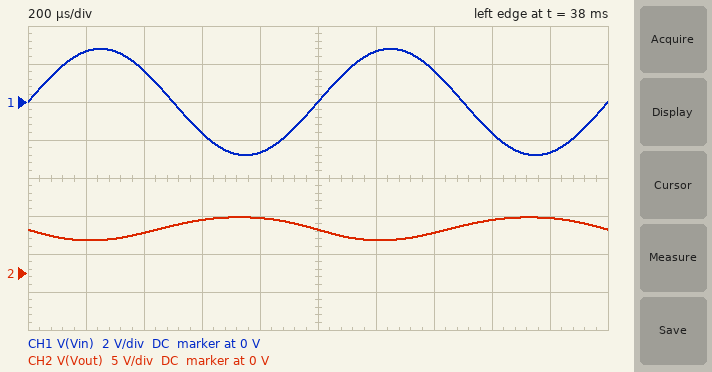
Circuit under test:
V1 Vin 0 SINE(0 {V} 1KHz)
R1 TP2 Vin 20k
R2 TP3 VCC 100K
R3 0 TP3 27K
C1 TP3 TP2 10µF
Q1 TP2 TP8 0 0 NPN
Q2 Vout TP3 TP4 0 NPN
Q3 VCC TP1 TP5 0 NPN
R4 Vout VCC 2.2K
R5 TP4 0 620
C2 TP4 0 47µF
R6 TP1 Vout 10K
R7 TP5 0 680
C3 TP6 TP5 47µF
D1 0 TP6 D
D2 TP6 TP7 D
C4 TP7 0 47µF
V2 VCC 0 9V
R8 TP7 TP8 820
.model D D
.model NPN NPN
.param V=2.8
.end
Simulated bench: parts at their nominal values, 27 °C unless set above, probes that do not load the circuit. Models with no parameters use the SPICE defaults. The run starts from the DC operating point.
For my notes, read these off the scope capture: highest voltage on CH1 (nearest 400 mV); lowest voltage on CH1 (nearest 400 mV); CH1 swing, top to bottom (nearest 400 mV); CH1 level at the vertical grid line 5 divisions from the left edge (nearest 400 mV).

2.8 V
-2.8 V
5.6 V
0 V
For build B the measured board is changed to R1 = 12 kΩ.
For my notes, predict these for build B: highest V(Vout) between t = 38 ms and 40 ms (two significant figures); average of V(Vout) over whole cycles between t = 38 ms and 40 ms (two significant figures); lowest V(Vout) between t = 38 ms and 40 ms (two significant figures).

7.5 V
5.9 V
4.2 V
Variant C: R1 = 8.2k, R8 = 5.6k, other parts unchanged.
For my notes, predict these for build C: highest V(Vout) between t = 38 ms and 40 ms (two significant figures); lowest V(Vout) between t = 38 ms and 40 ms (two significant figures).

8.7 V
2.7 V
